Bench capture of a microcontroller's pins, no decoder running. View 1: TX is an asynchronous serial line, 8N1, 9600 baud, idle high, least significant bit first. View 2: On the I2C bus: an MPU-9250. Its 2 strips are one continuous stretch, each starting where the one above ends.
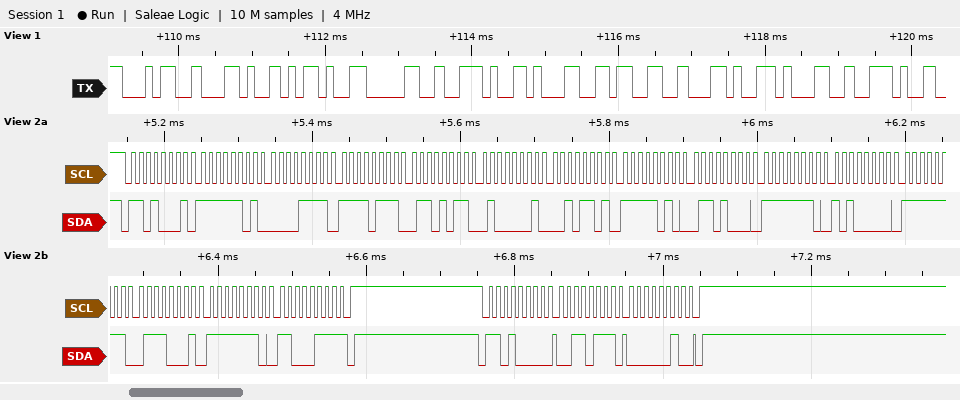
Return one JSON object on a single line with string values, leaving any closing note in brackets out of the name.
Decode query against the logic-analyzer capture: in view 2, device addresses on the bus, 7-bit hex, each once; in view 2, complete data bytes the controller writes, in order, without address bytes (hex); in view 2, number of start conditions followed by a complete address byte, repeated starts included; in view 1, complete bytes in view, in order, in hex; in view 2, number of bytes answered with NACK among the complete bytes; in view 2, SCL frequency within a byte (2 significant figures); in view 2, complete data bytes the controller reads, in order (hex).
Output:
{"in view 2, device addresses on the bus, 7-bit hex, each once": "0x68", "in view 2, complete data bytes the controller writes, in order, without address bytes": "37 02", "in view 2, number of start conditions followed by a complete address byte, repeated starts included": "2", "in view 1, complete bytes in view, in order, in hex": "0x34 0x2C 0x2D 0x30 0x2E 0x31 0x33 0x2C 0x31 0x2E", "in view 2, number of bytes answered with NACK among the complete bytes": "1", "in view 2, SCL frequency within a byte": "100 kHz", "in view 2, complete data bytes the controller reads, in order": "FD 0F F7 6B 41 2D FA 68 FE A0 FF 71 FE C7"}
